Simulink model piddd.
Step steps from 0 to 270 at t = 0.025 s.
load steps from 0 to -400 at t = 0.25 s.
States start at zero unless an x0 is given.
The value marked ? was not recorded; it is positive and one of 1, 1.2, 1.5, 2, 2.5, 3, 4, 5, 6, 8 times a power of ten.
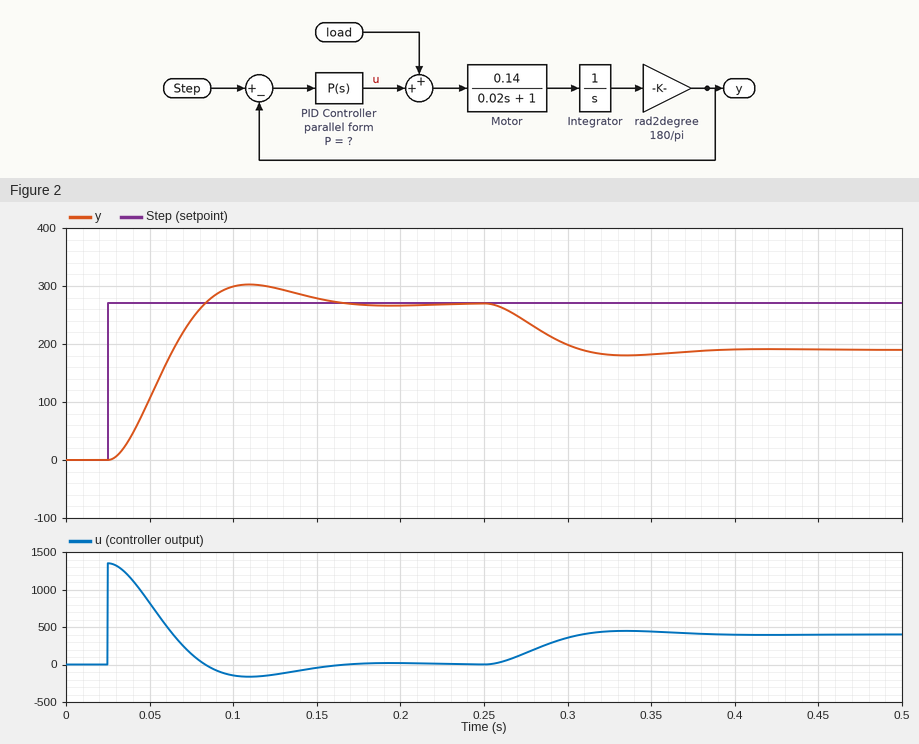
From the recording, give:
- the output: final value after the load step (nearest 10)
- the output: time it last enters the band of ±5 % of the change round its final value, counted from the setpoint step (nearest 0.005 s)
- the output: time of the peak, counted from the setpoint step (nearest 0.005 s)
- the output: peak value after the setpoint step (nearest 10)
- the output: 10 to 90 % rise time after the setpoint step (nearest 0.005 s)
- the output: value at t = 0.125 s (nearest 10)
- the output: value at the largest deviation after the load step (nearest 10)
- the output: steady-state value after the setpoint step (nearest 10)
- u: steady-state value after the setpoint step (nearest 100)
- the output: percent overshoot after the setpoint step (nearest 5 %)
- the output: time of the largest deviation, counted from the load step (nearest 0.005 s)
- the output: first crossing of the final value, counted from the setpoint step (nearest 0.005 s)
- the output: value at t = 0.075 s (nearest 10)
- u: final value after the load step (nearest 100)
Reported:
190
0.120 s
0.085 s
300
0.040 s
300
180
270
0
10 %
0.085 s
0.060 s
240
400
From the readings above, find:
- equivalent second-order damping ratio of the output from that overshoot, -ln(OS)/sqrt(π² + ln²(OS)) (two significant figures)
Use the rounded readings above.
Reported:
0.59
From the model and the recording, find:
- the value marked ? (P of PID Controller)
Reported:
5
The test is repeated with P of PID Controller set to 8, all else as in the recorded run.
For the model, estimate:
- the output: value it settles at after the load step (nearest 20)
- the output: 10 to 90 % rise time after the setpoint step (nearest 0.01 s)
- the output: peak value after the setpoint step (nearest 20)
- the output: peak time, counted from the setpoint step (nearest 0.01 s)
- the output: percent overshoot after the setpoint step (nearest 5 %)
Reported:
220
0.03 s
320
0.06 s
20 %
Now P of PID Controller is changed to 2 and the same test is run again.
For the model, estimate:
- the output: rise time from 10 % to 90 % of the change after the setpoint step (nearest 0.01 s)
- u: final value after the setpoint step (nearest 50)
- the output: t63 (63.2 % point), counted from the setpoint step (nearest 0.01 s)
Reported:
0.10 s
0
0.07 s
